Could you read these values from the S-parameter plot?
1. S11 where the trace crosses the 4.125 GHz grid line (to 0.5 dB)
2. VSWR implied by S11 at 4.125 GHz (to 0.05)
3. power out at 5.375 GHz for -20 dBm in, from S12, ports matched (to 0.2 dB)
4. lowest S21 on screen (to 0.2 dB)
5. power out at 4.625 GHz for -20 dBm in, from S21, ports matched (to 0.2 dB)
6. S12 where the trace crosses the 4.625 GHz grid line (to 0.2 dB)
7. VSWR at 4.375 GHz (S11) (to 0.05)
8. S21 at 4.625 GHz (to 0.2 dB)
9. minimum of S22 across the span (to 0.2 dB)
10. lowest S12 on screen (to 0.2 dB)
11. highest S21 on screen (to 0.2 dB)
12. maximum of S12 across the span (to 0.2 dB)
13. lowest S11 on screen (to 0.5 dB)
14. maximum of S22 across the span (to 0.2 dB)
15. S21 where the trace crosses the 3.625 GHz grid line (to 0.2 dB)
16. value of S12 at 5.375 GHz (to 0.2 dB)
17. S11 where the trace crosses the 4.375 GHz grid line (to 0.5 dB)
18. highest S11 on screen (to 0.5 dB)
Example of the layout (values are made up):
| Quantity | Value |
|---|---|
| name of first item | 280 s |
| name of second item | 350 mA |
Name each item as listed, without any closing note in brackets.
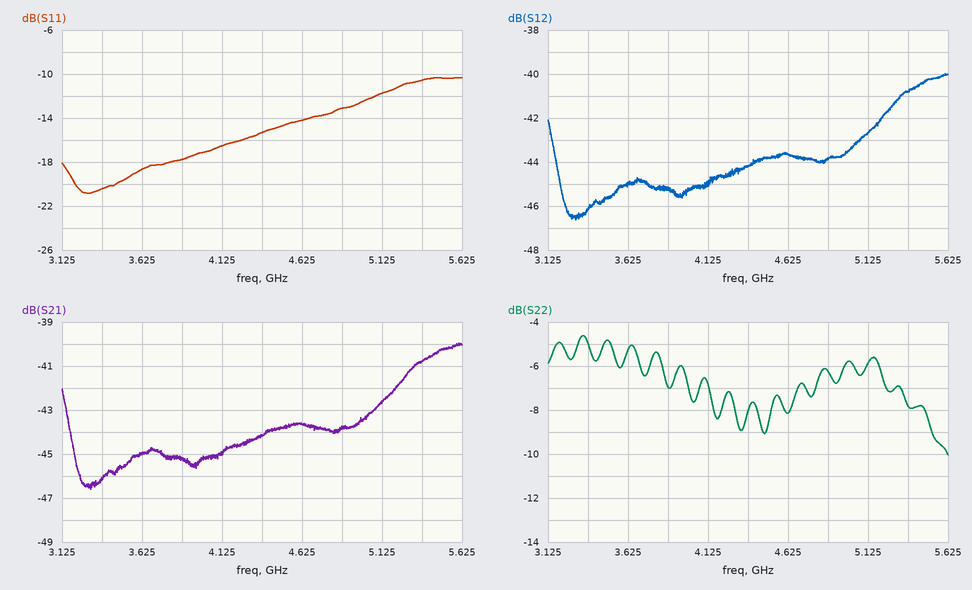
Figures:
| Quantity | Value |
|---|---|
| S11 where the trace crosses the 4.125 GHz grid line | -16.5 dB |
| VSWR implied by S11 at 4.125 GHz | 1.35 |
| power out at 5.375 GHz for -20 dBm in, from S12, ports matched | -60.8 dBm |
| lowest S21 on screen | -46.6 dB |
| power out at 4.625 GHz for -20 dBm in, from S21, ports matched | -63.6 dBm |
| S12 where the trace crosses the 4.625 GHz grid line | -43.6 dB |
| VSWR at 4.375 GHz (S11) | 1.40 |
| S21 at 4.625 GHz | -43.6 dB |
| minimum of S22 across the span | -10.0 dB |
| lowest S12 on screen | -46.6 dB |
| highest S21 on screen | -40.0 dB |
| maximum of S12 across the span | -40.0 dB |
| lowest S11 on screen | -21.0 dB |
| maximum of S22 across the span | -4.6 dB |
| S21 where the trace crosses the 3.625 GHz grid line | -45.0 dB |
| value of S12 at 5.375 GHz | -40.8 dB |
| S11 where the trace crosses the 4.375 GHz grid line | -15.5 dB |
| highest S11 on screen | -10.5 dB |
